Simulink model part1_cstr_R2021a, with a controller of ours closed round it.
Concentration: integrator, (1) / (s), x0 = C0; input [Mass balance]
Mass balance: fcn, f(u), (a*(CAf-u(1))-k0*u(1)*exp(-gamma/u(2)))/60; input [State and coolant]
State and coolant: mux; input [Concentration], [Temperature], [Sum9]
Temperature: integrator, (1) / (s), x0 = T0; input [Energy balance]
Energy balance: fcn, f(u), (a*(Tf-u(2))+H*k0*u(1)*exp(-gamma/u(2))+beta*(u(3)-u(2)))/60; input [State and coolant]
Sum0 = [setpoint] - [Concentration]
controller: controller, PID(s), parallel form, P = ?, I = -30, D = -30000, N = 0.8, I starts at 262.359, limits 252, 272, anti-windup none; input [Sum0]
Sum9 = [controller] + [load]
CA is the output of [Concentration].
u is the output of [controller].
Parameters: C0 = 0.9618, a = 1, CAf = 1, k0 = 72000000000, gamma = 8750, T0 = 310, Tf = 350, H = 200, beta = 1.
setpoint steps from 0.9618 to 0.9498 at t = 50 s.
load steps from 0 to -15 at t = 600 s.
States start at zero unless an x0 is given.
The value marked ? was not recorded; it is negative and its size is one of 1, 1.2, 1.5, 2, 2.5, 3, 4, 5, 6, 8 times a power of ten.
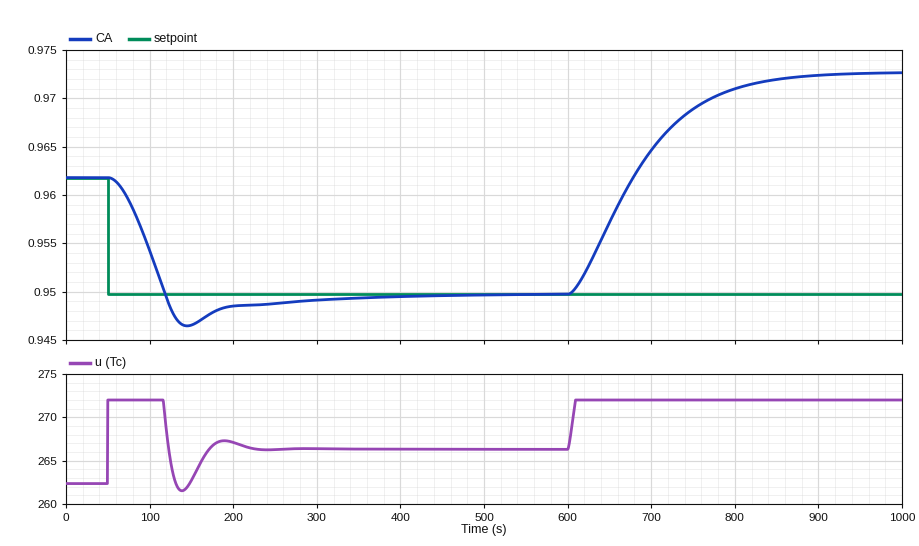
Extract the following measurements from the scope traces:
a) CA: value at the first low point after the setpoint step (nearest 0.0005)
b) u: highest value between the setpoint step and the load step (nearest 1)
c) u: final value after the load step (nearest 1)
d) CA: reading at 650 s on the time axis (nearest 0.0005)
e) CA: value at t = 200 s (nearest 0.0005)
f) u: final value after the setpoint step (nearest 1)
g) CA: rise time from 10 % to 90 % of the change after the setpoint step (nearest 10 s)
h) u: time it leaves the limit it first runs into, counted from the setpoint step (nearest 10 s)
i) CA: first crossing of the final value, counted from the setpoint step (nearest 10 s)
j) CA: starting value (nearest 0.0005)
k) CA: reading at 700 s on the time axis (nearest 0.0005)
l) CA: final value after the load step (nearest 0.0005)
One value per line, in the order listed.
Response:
0.9465
272
272
0.9570
0.9485
266
50 s
70 s
70 s
0.9620
0.9645
0.9725
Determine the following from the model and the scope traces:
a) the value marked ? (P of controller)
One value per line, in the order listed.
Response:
-4000
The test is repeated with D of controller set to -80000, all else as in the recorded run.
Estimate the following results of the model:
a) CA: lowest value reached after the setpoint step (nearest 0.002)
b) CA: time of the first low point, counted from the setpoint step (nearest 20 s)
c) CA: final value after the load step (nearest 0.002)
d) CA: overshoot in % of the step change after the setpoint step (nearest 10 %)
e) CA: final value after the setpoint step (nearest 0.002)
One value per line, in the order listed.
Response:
0.948
120 s
0.972
20 %
0.950
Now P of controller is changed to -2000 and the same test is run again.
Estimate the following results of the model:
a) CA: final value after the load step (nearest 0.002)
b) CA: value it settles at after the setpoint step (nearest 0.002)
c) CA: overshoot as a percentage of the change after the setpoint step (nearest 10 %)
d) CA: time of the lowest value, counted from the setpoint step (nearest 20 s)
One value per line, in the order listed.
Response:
0.972
0.950
40 %
100 s
